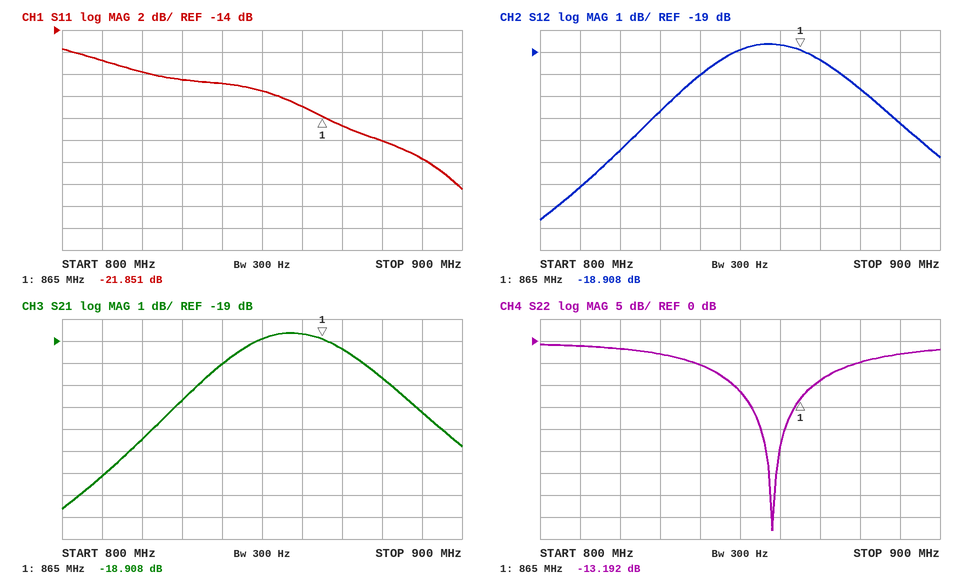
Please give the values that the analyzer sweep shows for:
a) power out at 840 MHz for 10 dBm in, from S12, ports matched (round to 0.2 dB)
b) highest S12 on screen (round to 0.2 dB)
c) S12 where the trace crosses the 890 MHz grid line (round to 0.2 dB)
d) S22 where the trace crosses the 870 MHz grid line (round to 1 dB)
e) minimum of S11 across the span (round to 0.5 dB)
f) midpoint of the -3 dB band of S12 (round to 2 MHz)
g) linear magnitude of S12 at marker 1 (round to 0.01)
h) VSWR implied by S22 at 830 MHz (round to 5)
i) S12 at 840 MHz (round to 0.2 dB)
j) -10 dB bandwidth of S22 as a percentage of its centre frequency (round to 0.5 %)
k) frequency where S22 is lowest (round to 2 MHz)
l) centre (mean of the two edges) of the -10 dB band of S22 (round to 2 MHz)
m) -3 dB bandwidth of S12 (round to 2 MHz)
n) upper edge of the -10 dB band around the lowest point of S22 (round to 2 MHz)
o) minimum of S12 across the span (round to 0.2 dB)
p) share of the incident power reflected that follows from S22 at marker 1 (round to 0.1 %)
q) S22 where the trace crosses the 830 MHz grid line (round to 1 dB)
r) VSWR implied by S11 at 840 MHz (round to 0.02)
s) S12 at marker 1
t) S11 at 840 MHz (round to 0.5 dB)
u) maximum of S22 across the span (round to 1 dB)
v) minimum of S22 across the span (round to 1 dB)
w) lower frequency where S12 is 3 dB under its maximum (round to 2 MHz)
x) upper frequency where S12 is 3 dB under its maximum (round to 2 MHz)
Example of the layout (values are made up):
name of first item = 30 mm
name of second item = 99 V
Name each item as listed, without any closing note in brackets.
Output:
power out at 840 MHz for 10 dBm in, from S12, ports matched = -10.0 dBm
highest S12 on screen = -18.6 dB
S12 where the trace crosses the 890 MHz grid line = -22.2 dB
S22 where the trace crosses the 870 MHz grid line = -9 dB
minimum of S11 across the span = -28.5 dB
midpoint of the -3 dB band of S12 = 858 MHz
linear magnitude of S12 at marker 1 = 0.11
VSWR implied by S22 at 830 MHz = 5
S12 at 840 MHz = -20.0 dB
-10 dB bandwidth of S22 as a percentage of its centre frequency = 2.5 %
frequency where S22 is lowest = 858 MHz
centre (mean of the two edges) of the -10 dB band of S22 = 858 MHz
-3 dB bandwidth of S12 = 56 MHz
upper edge of the -10 dB band around the lowest point of S22 = 868 MHz
minimum of S12 across the span = -26.6 dB
share of the incident power reflected that follows from S22 at marker 1 = 4.8 %
S22 where the trace crosses the 830 MHz grid line = -3 dB
VSWR implied by S11 at 840 MHz = 1.26
S12 at marker 1 = -18.908 dB
S11 at 840 MHz = -19.0 dB
maximum of S22 across the span = -1 dB
minimum of S22 across the span = -43 dB
lower frequency where S12 is 3 dB under its maximum = 830 MHz
upper frequency where S12 is 3 dB under its maximum = 886 MHz
